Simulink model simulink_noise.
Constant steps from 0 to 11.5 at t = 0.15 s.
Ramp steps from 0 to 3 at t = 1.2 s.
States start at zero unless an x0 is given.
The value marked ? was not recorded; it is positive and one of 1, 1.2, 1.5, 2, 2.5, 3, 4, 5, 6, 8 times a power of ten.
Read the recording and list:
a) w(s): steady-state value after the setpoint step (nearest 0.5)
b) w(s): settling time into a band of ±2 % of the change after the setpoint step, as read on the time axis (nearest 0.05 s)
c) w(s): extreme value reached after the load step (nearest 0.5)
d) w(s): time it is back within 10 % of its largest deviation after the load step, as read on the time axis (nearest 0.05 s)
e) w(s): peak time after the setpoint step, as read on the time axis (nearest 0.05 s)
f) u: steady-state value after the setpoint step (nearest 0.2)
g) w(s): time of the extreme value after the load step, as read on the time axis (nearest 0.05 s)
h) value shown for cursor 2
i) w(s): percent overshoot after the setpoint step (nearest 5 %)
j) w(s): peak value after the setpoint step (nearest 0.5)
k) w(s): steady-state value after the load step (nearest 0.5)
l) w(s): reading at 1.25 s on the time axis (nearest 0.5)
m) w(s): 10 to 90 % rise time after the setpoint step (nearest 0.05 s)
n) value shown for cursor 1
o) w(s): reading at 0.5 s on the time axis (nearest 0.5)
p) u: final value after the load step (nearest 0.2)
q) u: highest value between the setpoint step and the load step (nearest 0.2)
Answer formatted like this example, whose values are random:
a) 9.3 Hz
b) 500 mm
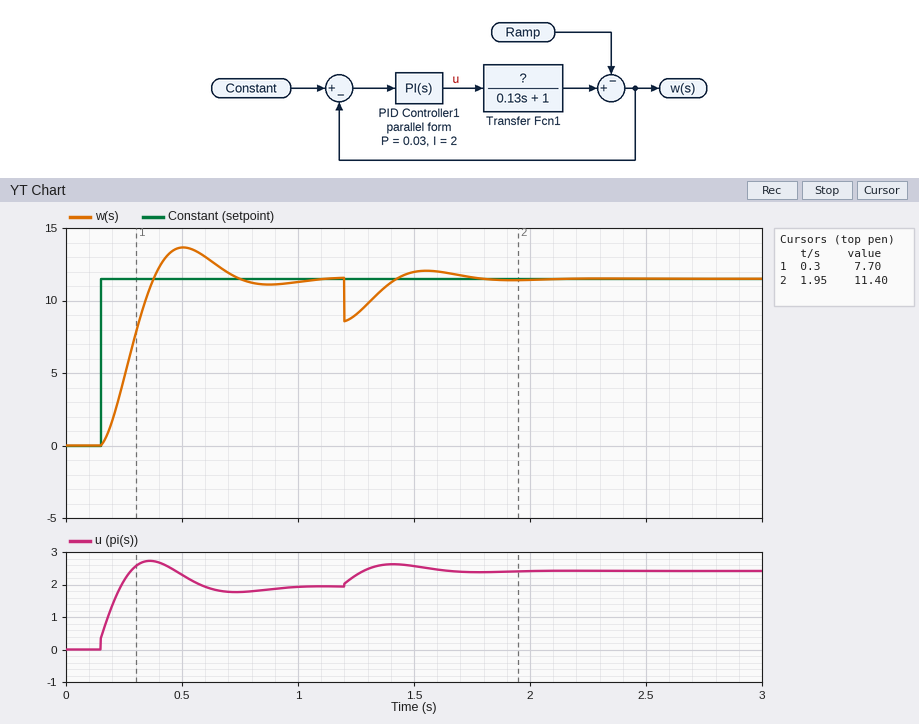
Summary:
a) 11.5
b) 1.00 s
c) 8.5
d) 1.70 s
e) 0.50 s
f) 2.0
g) 1.20 s
h) 11.40
i) 20 %
j) 13.5
k) 11.5
l) 9.0
m) 0.15 s
n) 7.70
o) 13.5
p) 2.4
q) 2.8
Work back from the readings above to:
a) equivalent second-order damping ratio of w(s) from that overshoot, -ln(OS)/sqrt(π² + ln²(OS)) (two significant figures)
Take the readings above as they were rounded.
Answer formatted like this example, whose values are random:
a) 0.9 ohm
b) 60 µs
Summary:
a) 0.46
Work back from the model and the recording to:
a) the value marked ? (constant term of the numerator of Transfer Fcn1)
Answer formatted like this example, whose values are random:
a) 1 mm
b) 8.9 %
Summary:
a) 6
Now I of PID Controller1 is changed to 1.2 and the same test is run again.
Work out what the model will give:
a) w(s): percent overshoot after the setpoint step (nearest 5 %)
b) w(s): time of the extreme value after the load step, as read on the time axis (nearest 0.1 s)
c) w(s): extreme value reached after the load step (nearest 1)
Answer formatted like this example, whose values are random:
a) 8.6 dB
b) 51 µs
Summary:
a) 10 %
b) 1.2 s
c) 8
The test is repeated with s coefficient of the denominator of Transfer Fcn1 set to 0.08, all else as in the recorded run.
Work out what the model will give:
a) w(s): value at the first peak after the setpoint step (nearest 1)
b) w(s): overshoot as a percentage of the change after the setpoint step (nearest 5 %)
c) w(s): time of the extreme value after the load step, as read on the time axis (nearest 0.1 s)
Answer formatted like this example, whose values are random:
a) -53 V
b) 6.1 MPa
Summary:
a) 13
b) 10 %
c) 1.2 s
